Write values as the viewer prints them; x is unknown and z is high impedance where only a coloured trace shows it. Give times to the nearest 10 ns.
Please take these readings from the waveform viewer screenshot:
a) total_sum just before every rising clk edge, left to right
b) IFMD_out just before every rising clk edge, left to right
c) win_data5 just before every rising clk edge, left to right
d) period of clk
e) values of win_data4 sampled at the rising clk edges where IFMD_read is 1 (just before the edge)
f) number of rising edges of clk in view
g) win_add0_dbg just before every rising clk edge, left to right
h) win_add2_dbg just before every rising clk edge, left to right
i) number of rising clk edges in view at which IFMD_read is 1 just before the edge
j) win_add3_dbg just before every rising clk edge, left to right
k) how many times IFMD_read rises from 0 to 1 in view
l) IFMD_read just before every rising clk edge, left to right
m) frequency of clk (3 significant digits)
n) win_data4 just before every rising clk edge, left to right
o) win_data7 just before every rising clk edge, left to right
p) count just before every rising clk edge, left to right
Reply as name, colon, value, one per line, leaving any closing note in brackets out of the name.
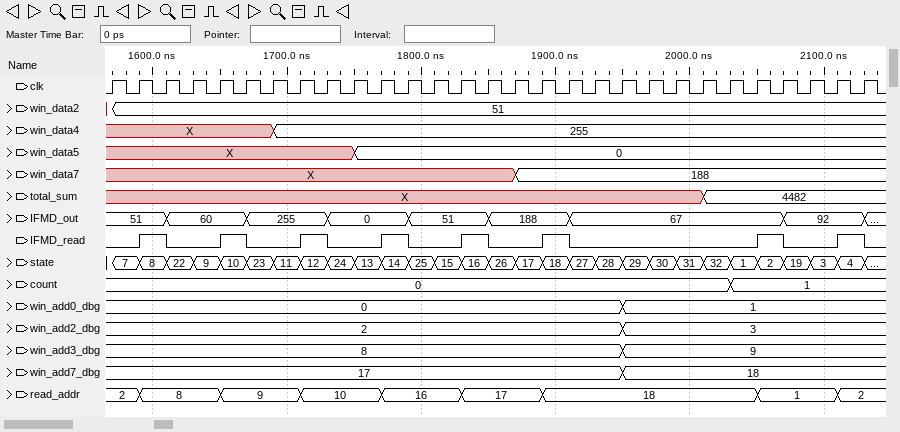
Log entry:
total_sum just before every rising clk edge, left to right: X, X, X, X, X, X, X, X, X, X, X, X, X, X, X, X, X, X, X, X, X, X, X, 4482, 4482, 4482, 4482, 4482, 4482
IFMD_out just before every rising clk edge, left to right: 51, 51, 51, 60, 60, 60, 255, 255, 255, 0, 0, 0, 51, 51, 51, 188, 188, 188, 67, 67, 67, 67, 67, 67, 67, 67, 92, 92, 92
win_data5 just before every rising clk edge, left to right: X, X, X, X, X, X, X, X, X, X, 0, 0, 0, 0, 0, 0, 0, 0, 0, 0, 0, 0, 0, 0, 0, 0, 0, 0, 0
period of clk: 20 ns
values of win_data4 sampled at the rising clk edges where IFMD_read is 1: X, X, 255, 255, 255, 255, 255, 255
number of rising edges of clk in view: 29
win_add0_dbg just before every rising clk edge, left to right: 0, 0, 0, 0, 0, 0, 0, 0, 0, 0, 0, 0, 0, 0, 0, 0, 0, 0, 0, 0, 1, 1, 1, 1, 1, 1, 1, 1, 1
win_add2_dbg just before every rising clk edge, left to right: 2, 2, 2, 2, 2, 2, 2, 2, 2, 2, 2, 2, 2, 2, 2, 2, 2, 2, 2, 2, 3, 3, 3, 3, 3, 3, 3, 3, 3
number of rising clk edges in view at which IFMD_read is 1 just before the edge: 8
win_add3_dbg just before every rising clk edge, left to right: 8, 8, 8, 8, 8, 8, 8, 8, 8, 8, 8, 8, 8, 8, 8, 8, 8, 8, 8, 8, 9, 9, 9, 9, 9, 9, 9, 9, 9
how many times IFMD_read rises from 0 to 1 in view: 8
IFMD_read just before every rising clk edge, left to right: 0 0 1 0 0 1 0 0 1 0 0 1 0 0 1 0 0 1 0 0 0 0 0 0 0 1 0 0 1
frequency of clk: 50.0 MHz
win_data4 just before every rising clk edge, left to right: X, X, X, X, X, X, X, 255, 255, 255, 255, 255, 255, 255, 255, 255, 255, 255, 255, 255, 255, 255, 255, 255, 255, 255, 255, 255, 255
win_data7 just before every rising clk edge, left to right: X, X, X, X, X, X, X, X, X, X, X, X, X, X, X, X, 188, 188, 188, 188, 188, 188, 188, 188, 188, 188, 188, 188, 188
count just before every rising clk edge, left to right: 0, 0, 0, 0, 0, 0, 0, 0, 0, 0, 0, 0, 0, 0, 0, 0, 0, 0, 0, 0, 0, 0, 0, 0, 1, 1, 1, 1, 1
